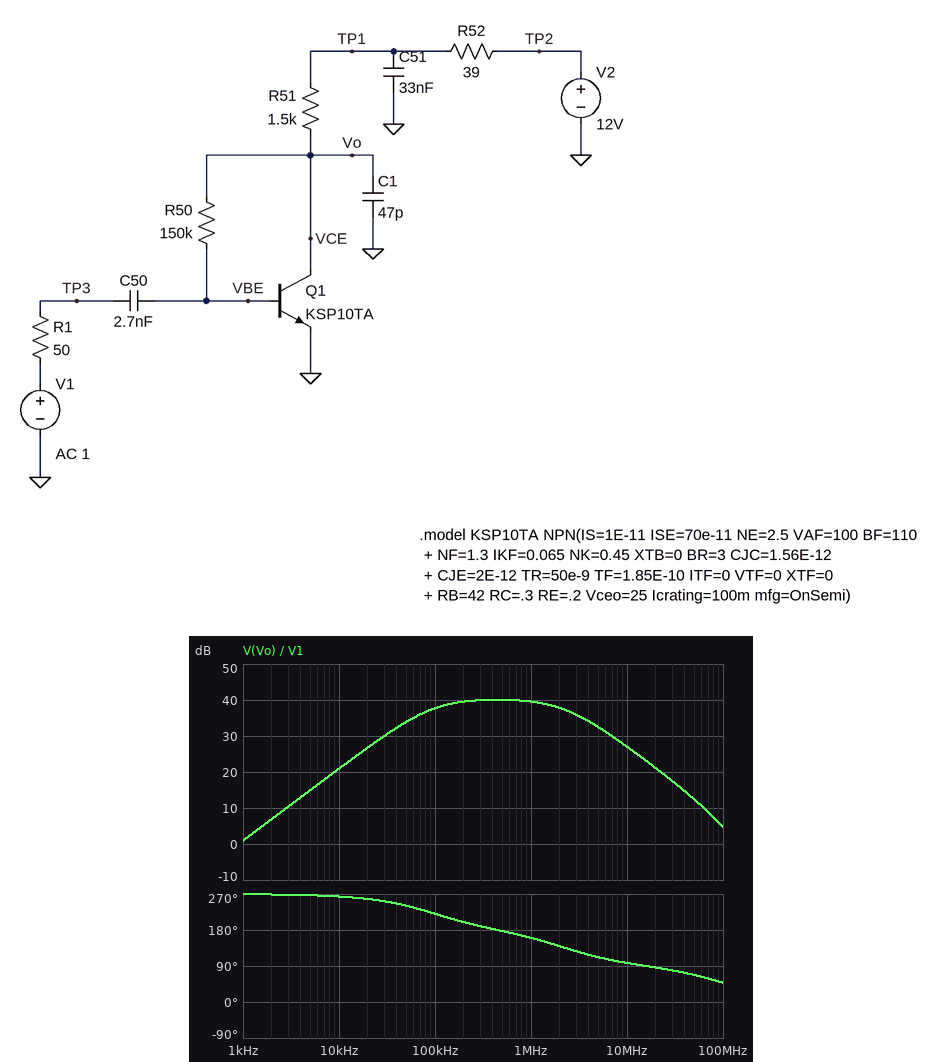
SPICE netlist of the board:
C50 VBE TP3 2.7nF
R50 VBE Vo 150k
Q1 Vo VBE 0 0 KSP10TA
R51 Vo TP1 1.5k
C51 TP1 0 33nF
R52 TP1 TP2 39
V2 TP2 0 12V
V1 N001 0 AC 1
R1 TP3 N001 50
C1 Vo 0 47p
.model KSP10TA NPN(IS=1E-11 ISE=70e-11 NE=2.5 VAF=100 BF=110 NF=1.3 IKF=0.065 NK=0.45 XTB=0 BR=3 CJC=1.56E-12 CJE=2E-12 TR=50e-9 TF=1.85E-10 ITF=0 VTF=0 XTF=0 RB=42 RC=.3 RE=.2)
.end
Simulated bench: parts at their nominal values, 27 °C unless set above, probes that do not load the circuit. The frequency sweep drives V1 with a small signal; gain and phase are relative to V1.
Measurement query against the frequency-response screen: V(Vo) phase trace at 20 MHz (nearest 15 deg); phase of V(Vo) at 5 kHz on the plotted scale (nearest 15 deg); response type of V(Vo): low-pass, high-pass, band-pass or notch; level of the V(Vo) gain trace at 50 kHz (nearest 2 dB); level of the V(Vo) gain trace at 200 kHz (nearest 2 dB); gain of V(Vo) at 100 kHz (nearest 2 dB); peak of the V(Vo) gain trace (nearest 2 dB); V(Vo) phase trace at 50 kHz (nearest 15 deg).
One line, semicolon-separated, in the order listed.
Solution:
90 deg; 270 deg; band-pass; 34 dB; 40 dB; 38 dB; 40 dB; 240 deg
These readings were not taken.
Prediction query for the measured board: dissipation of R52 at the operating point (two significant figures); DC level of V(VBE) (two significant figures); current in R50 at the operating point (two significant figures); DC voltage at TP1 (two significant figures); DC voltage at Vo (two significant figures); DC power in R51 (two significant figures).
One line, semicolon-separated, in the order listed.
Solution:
360 µW; 660 mV; 44 µA; 12 V; 7.3 V; 14 mW
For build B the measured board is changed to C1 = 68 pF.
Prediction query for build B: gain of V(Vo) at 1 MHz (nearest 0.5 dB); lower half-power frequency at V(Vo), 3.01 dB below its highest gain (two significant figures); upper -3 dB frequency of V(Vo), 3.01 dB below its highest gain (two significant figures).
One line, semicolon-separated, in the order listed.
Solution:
39.0 dB; 84 kHz; 1.7 MHz
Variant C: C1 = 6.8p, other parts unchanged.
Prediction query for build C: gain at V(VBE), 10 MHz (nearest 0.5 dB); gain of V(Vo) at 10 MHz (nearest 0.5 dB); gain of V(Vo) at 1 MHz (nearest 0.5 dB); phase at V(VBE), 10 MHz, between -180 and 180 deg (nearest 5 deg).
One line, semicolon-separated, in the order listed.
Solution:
-2.0 dB; 37.0 dB; 40.0 dB; -5 deg
